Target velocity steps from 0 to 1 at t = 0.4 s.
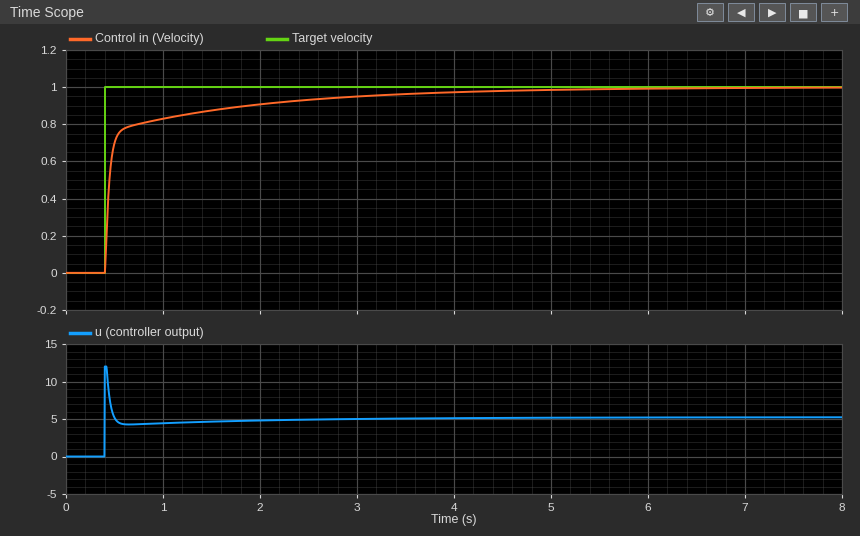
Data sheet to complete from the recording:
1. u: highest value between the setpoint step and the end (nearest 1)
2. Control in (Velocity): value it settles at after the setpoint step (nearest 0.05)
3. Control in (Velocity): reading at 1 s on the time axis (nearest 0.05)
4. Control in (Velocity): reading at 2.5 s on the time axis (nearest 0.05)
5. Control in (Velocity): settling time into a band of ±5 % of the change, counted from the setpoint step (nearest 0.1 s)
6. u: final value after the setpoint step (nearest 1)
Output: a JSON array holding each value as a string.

["12", "1.00", "0.85", "0.95", "2.6 s", "5"]
